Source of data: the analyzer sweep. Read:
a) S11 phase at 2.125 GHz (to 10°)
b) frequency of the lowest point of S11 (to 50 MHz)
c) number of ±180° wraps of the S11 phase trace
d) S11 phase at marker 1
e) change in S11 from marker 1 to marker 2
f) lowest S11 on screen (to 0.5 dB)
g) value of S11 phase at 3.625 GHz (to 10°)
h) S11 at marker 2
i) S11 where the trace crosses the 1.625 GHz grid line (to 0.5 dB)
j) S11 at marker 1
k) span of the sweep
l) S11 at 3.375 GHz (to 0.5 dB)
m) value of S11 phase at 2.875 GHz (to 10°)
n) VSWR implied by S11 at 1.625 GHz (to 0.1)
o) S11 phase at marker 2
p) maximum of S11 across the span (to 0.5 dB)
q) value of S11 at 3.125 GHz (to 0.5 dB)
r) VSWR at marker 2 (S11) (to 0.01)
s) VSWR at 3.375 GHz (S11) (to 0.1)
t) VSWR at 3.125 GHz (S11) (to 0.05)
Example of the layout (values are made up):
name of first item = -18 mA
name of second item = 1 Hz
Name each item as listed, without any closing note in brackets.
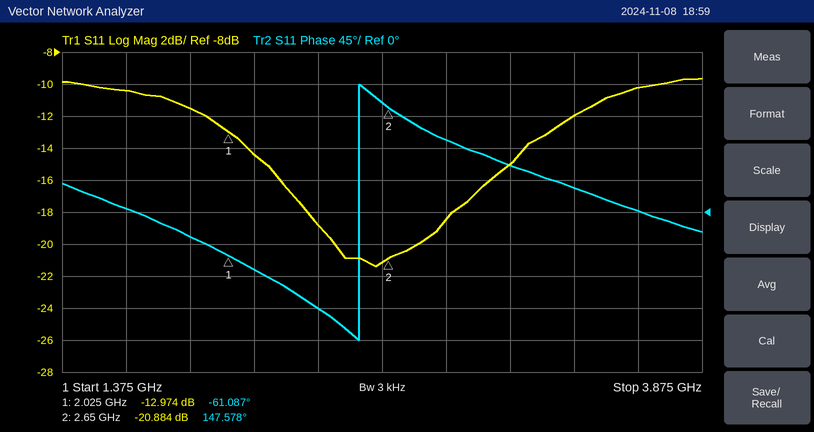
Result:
S11 phase at 2.125 GHz = -80°
frequency of the lowest point of S11 = 2.60 GHz
number of ±180° wraps of the S11 phase trace = 1
S11 phase at marker 1 = -61.087°
change in S11 from marker 1 to marker 2 = -7.910 dB
lowest S11 on screen = -21.5 dB
value of S11 phase at 3.625 GHz = 0°
S11 at marker 2 = -20.884 dB
S11 where the trace crosses the 1.625 GHz grid line = -10.5 dB
S11 at marker 1 = -12.974 dB
span of the sweep = 2.5 GHz
S11 at 3.375 GHz = -12.0 dB
value of S11 phase at 2.875 GHz = 100°
VSWR implied by S11 at 1.625 GHz = 1.9
S11 phase at marker 2 = 147.578°
maximum of S11 across the span = -9.5 dB
value of S11 at 3.125 GHz = -15.0 dB
VSWR at marker 2 (S11) = 1.20
VSWR at 3.375 GHz (S11) = 1.7
VSWR at 3.125 GHz (S11) = 1.45
